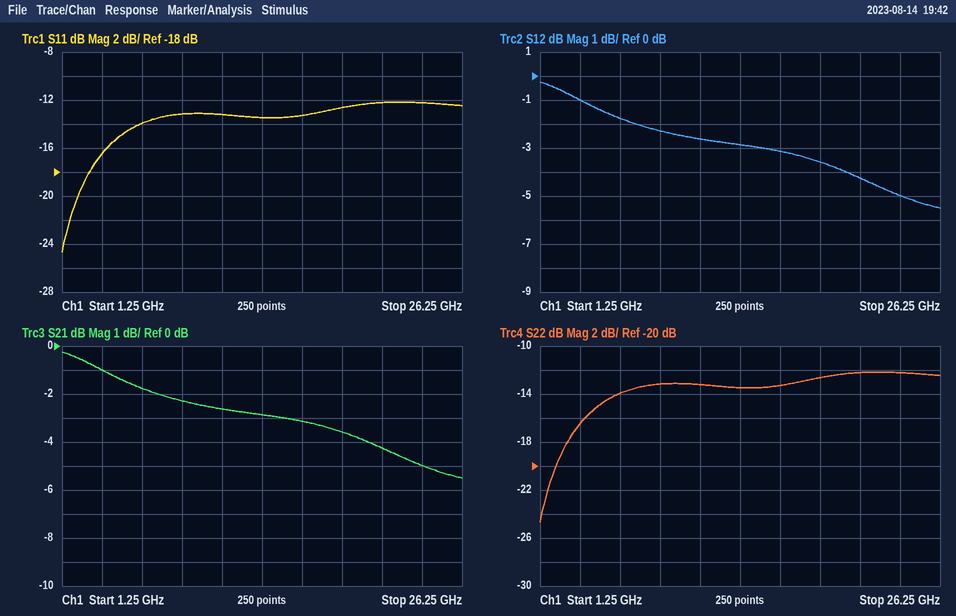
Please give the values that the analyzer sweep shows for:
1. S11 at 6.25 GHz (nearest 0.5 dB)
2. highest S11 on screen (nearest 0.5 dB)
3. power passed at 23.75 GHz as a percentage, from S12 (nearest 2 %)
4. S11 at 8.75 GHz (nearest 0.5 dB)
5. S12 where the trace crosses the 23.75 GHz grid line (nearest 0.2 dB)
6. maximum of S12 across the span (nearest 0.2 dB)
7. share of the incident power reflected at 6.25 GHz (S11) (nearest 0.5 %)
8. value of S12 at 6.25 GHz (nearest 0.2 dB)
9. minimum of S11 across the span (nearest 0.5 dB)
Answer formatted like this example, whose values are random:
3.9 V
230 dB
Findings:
-14.0 dB
-12.0 dB
32 %
-13.0 dB
-5.0 dB
-0.2 dB
4.0 %
-1.8 dB
-24.5 dB
